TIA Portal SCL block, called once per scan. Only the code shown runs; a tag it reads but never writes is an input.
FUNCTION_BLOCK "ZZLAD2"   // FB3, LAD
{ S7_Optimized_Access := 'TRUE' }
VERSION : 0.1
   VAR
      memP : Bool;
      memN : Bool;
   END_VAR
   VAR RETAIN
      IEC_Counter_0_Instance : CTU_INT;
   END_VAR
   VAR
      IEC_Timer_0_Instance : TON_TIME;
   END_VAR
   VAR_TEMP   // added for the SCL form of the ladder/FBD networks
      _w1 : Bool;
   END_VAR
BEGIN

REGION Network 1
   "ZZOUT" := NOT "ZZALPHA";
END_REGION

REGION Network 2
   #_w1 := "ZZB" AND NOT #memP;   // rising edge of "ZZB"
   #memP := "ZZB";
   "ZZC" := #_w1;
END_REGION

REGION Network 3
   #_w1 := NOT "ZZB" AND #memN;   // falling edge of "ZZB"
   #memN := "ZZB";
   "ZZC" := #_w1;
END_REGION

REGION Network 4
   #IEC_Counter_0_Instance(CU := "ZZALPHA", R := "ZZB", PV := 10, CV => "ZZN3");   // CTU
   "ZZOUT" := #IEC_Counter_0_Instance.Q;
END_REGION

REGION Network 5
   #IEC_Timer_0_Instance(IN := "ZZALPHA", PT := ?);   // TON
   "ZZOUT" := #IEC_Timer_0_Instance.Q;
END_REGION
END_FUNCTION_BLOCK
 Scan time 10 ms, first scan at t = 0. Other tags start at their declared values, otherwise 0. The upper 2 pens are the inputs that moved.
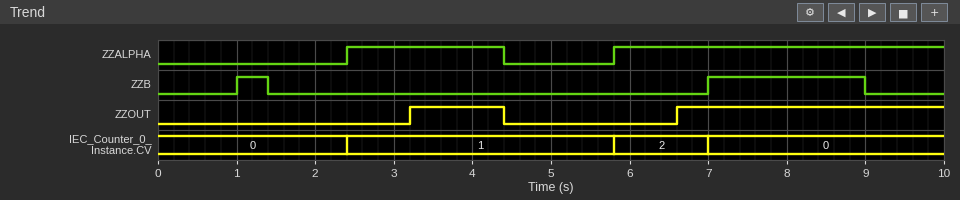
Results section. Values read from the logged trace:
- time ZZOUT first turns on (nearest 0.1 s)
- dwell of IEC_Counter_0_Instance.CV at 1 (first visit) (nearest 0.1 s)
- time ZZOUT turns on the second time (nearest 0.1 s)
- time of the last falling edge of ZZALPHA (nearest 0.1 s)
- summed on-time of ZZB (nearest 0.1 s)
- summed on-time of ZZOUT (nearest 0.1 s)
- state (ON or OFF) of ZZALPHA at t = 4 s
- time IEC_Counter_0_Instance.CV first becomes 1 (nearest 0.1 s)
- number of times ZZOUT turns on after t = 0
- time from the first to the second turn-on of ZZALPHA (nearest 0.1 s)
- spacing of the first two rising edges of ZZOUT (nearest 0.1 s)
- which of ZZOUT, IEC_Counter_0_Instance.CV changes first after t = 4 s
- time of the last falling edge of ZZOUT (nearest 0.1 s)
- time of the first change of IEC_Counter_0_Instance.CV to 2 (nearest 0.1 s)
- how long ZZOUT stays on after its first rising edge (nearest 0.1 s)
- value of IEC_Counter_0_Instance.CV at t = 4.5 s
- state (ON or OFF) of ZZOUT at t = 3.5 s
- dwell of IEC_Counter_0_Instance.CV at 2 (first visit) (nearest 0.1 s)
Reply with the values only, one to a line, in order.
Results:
3.2 s
3.4 s
6.6 s
4.4 s
2.4 s
4.6 s
ON
2.4 s
2
3.4 s
3.4 s
ZZOUT
4.4 s
5.8 s
1.2 s
1
ON
1.2 s
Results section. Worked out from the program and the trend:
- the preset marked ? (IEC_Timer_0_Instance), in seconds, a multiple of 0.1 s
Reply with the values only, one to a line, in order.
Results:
0.8 s
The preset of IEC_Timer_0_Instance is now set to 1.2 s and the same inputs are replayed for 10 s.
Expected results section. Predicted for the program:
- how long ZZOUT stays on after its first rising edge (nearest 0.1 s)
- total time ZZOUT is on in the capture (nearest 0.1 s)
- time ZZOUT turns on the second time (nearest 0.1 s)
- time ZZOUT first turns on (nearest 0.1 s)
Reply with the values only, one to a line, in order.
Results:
0.8 s
3.8 s
7.0 s
3.6 s
